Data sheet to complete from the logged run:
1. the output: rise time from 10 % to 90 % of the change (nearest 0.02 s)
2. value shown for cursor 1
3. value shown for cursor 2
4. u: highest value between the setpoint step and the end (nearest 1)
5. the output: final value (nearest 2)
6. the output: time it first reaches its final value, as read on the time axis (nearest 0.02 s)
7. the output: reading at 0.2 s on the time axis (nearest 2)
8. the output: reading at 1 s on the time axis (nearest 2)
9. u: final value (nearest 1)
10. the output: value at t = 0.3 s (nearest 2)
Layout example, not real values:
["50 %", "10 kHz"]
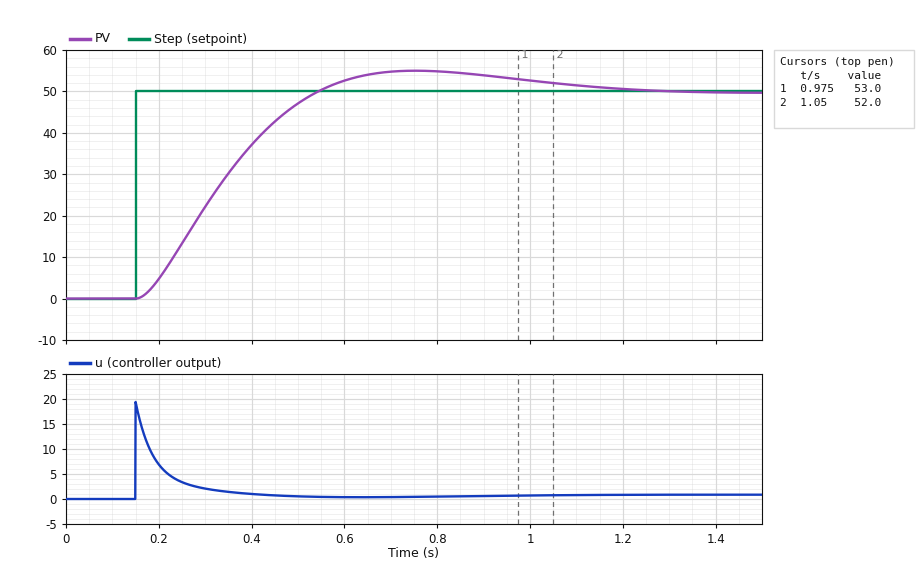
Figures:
["0.28 s", "53.0", "52.0", "19", "50", "0.54 s", "4", "52", "1", "22"]
